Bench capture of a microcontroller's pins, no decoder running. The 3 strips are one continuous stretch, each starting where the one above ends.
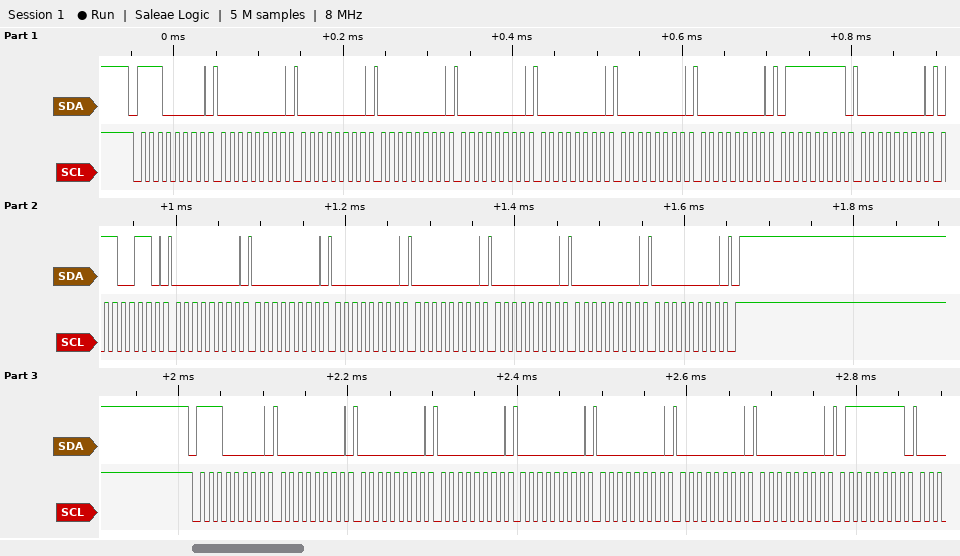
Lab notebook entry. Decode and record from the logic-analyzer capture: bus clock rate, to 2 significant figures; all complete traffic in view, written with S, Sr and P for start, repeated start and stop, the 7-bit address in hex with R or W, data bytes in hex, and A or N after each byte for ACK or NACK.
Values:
100 kHz
S 70W A 00 A 00 A 00 A 00 A 00 A 00 A 00 A 7F A 00 A 66 A 00 A 00 A 00 A 00 A 00 A 00 A 00 A P S 70W A 00 A 00 A 00 A 00 A 00 A 00 A 00 A 7F A
